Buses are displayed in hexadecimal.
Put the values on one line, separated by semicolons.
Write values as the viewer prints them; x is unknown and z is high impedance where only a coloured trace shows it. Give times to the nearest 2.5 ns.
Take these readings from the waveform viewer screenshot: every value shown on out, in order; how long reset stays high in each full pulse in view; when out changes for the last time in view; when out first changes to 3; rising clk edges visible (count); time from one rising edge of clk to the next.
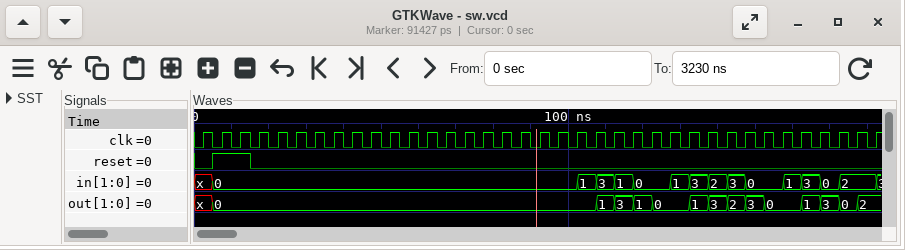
x, 0, 1, 3, 1, 0, 1, 3, 2, 3, 0, 1, 3, 0, 2; 10 ns; 177.5 ns; 112.5 ns; 37; 5 ns
